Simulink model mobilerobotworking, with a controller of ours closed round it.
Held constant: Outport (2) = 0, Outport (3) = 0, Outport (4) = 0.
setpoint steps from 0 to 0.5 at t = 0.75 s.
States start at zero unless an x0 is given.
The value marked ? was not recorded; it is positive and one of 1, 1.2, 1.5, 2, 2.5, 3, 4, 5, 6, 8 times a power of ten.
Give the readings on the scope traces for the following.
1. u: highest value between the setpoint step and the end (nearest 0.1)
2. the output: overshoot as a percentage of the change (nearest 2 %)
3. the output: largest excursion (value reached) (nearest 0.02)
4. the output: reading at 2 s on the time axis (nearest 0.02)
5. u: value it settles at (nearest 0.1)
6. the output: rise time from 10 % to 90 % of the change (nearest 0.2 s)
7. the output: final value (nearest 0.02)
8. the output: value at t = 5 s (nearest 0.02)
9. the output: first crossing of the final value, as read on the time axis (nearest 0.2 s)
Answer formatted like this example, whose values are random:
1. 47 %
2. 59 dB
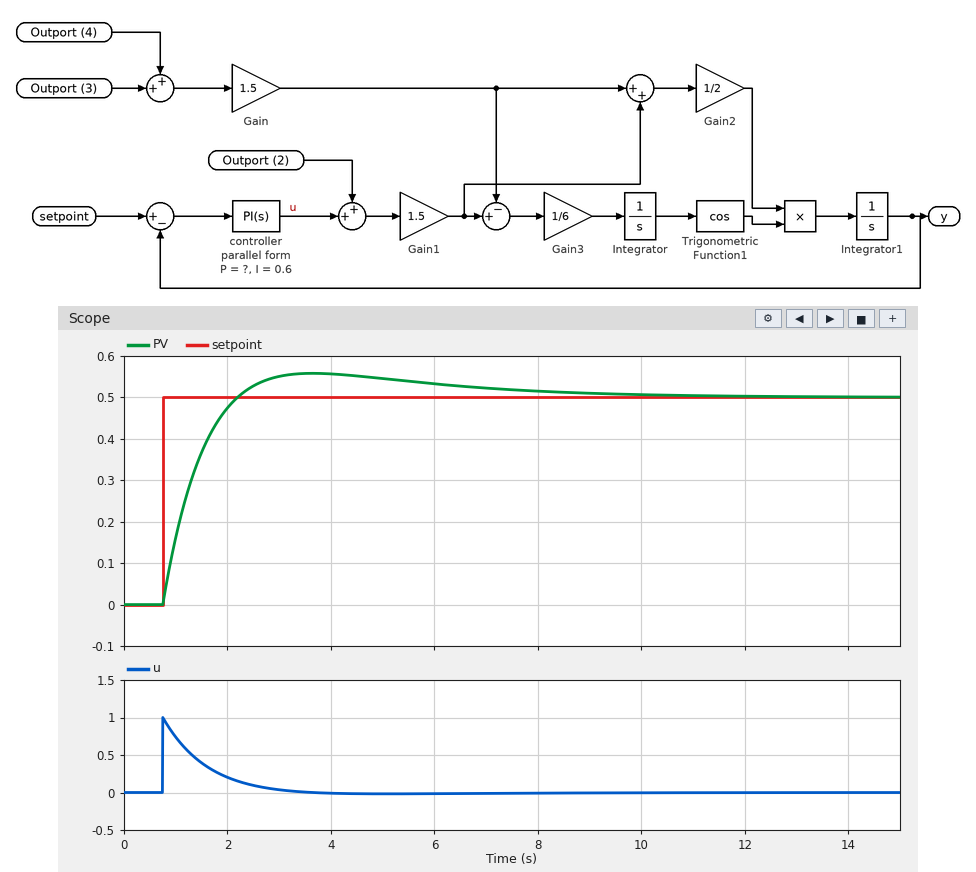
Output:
1. 1.0
2. 12 %
3. 0.56
4. 0.48
5. 0.0
6. 1.0 s
7. 0.50
8. 0.54
9. 2.2 s
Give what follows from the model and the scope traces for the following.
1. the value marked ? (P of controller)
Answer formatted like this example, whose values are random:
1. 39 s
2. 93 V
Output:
1. 2
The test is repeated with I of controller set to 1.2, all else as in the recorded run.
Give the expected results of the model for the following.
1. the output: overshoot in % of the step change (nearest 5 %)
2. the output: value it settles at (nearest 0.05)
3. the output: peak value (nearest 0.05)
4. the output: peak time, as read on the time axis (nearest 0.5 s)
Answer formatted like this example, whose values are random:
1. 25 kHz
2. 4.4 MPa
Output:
1. 20 %
2. 0.50
3. 0.60
4. 3.0 s
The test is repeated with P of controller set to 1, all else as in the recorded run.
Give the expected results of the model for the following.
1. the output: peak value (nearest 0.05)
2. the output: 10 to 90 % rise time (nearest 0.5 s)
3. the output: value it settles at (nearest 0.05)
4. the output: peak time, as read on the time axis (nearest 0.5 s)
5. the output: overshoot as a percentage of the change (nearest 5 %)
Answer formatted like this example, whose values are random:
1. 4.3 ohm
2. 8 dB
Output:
1. 0.65
2. 1.5 s
3. 0.50
4. 4.5 s
5. 25 %
